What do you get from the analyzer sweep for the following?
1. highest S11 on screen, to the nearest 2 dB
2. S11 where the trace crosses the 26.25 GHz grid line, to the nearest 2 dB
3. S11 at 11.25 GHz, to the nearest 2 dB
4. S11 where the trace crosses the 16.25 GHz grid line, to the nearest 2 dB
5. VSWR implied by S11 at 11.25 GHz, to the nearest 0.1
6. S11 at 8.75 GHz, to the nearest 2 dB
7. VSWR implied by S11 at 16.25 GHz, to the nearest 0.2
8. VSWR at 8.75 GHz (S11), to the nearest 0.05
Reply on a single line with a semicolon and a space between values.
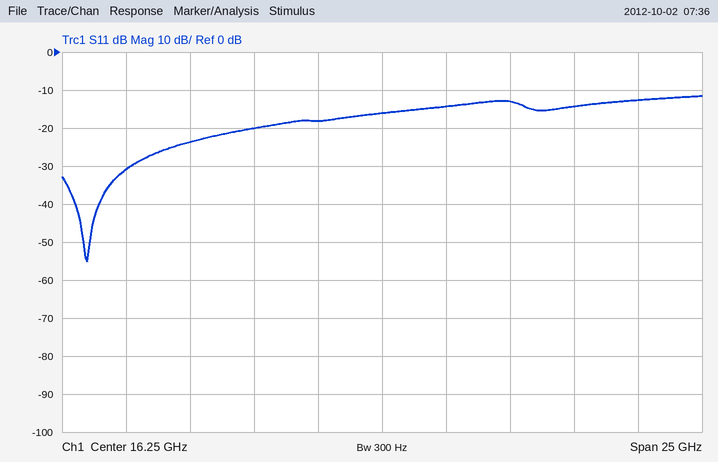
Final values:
-12 dB; -12 dB; -20 dB; -16 dB; 1.2; -24 dB; 1.4; 1.15
